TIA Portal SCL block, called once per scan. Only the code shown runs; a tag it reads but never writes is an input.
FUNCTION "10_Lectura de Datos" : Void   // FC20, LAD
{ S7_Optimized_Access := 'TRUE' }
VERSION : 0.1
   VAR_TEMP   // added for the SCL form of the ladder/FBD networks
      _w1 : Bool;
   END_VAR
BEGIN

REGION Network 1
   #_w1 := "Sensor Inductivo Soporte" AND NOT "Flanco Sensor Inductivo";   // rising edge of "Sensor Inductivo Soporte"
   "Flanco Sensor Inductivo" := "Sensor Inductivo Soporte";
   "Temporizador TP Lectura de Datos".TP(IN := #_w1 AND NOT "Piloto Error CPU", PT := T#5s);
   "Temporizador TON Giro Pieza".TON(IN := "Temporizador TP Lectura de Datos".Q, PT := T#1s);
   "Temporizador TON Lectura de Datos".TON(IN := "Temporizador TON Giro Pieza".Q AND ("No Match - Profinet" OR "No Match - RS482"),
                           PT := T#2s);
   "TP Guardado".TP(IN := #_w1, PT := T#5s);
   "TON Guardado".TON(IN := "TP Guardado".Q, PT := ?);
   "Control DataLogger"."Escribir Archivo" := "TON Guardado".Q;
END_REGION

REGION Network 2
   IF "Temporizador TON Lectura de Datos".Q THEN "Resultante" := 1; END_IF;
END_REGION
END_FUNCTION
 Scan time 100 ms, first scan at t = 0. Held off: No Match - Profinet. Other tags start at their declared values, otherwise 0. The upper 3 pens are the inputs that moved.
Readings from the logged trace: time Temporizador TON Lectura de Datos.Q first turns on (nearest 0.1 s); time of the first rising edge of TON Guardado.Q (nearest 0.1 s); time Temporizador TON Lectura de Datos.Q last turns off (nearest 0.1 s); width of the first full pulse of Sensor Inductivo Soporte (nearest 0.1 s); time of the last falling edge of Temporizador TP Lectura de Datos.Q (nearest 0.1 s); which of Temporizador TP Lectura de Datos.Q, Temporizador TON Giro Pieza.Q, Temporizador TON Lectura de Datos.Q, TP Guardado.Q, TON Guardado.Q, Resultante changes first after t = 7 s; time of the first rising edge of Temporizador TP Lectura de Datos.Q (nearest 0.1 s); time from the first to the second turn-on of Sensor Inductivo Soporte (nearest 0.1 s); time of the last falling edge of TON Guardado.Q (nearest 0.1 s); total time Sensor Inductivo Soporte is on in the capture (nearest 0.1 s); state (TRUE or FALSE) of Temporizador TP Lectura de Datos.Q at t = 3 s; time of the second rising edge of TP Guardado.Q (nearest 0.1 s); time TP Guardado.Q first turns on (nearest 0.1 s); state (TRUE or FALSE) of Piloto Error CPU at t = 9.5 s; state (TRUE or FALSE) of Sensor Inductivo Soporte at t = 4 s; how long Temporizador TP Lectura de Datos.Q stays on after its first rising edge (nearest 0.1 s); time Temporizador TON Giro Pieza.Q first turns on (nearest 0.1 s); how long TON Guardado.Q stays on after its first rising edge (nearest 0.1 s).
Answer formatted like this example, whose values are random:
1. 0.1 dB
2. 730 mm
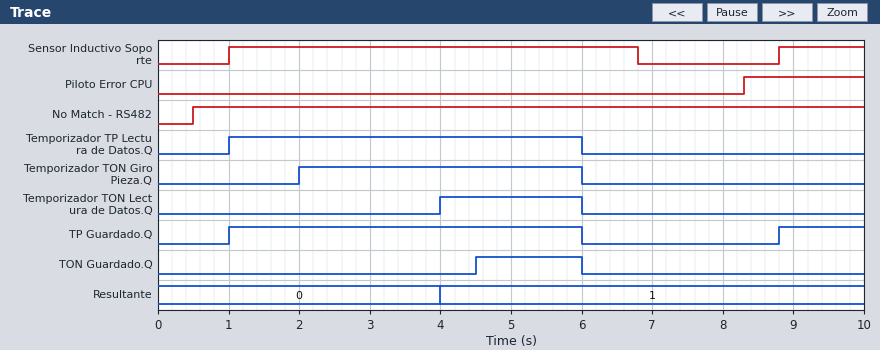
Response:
1. 4.0 s
2. 4.5 s
3. 6.0 s
4. 5.8 s
5. 6.0 s
6. TP Guardado.Q
7. 1.0 s
8. 7.8 s
9. 6.0 s
10. 7.0 s
11. TRUE
12. 8.8 s
13. 1.0 s
14. TRUE
15. TRUE
16. 5.0 s
17. 2.0 s
18. 1.5 s
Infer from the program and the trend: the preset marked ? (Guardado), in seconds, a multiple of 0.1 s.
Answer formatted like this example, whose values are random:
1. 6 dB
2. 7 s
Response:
1. 3.5 s
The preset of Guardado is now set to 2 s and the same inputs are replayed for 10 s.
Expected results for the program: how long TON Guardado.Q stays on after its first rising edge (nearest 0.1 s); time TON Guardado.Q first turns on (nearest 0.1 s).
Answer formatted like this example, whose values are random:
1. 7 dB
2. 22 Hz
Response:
1. 3.0 s
2. 3.0 s
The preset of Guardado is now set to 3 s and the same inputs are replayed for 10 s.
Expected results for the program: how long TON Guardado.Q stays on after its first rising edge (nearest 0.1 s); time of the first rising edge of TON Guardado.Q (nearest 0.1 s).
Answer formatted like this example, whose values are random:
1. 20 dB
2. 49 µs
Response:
1. 2.0 s
2. 4.0 s
